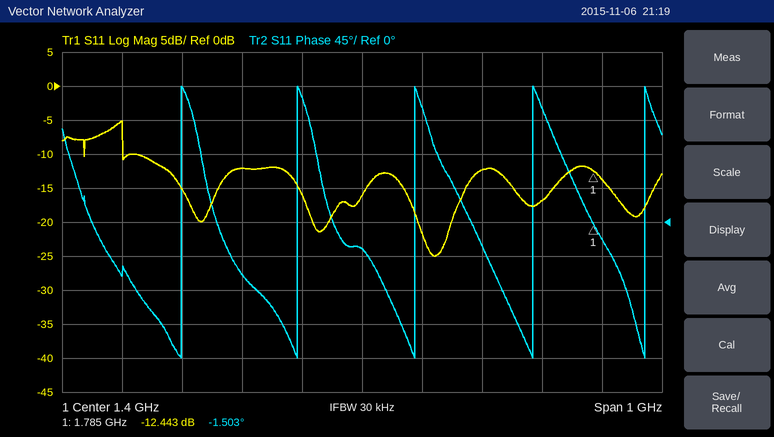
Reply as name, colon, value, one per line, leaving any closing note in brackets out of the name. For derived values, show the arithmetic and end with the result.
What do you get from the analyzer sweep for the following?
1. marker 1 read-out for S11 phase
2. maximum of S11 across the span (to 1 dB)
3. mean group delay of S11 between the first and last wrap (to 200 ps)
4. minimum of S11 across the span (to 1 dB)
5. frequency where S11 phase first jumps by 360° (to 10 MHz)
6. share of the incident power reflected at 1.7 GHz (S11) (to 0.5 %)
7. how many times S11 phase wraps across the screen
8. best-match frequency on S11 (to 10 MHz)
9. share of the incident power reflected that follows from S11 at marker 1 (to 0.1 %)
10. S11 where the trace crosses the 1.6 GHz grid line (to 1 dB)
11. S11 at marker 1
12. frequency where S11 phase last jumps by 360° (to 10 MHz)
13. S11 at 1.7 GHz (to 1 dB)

marker 1 read-out for S11 phase: -1.503°
maximum of S11 across the span: -5 dB
mean group delay of S11 between the first and last wrap: 4 cycles / (1.87 GHz − 1.10 GHz) ≈ 5.2 ns
minimum of S11 across the span: -25 dB
frequency where S11 phase first jumps by 360°: 1.10 GHz
share of the incident power reflected at 1.7 GHz (S11): 10^(-17/10) ≈ 2.0 %
how many times S11 phase wraps across the screen: 5
best-match frequency on S11: 1.52 GHz
share of the incident power reflected that follows from S11 at marker 1: 10^(-12.443/10) ≈ 5.7 %
S11 where the trace crosses the 1.6 GHz grid line: -12 dB
S11 at marker 1: -12.443 dB
frequency where S11 phase last jumps by 360°: 1.87 GHz
S11 at 1.7 GHz: -17 dB
